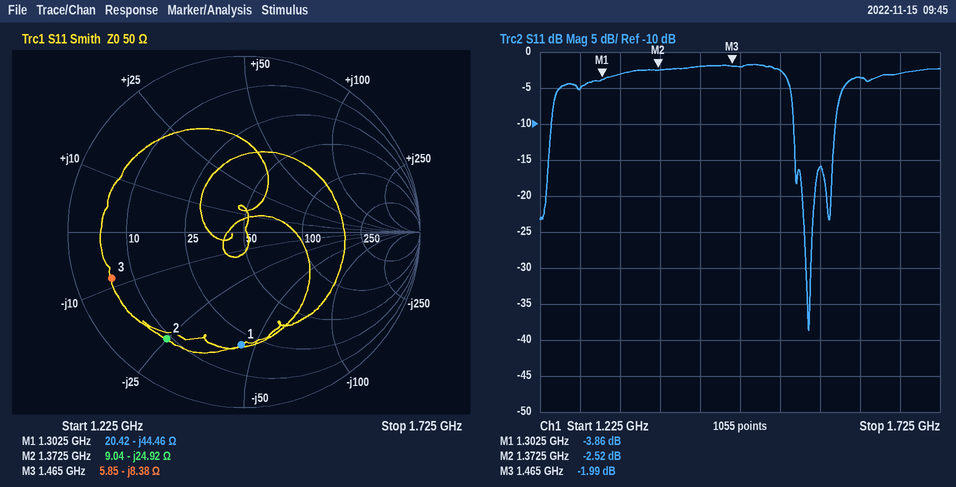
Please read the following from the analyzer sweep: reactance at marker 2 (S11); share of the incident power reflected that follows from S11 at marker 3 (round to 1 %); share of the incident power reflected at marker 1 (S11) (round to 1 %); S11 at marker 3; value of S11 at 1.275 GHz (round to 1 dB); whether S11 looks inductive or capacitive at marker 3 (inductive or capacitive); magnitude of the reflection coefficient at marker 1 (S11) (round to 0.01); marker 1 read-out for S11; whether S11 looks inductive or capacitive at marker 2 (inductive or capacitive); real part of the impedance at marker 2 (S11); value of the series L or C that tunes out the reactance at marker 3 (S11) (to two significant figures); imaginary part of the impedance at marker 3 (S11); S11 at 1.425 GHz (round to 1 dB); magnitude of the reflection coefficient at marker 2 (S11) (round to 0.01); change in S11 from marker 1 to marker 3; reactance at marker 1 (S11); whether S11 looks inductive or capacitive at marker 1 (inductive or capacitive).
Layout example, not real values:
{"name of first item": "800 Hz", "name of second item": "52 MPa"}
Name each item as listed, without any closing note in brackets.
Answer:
{"reactance at marker 2": "-24.92 Ω", "share of the incident power reflected that follows from S11 at marker 3": "63 %", "share of the incident power reflected at marker 1 (S11)": "41 %", "S11 at marker 3": "-1.99 dB", "value of S11 at 1.275 GHz": "-5 dB", "whether S11 looks inductive or capacitive at marker 3": "capacitive", "magnitude of the reflection coefficient at marker 1 (S11)": "0.64", "marker 1 read-out for S11": "-3.86 dB", "whether S11 looks inductive or capacitive at marker 2": "capacitive", "real part of the impedance at marker 2": "9.04 Ω", "value of the series L or C that tunes out the reactance at marker 3 (S11)": "910 pH", "imaginary part of the impedance at marker 3": "-8.38 Ω", "S11 at 1.425 GHz": "-2 dB", "magnitude of the reflection coefficient at marker 2 (S11)": "0.75", "change in S11 from marker 1 to marker 3": "1.87 dB", "reactance at marker 1": "-44.46 Ω", "whether S11 looks inductive or capacitive at marker 1": "capacitive"}
